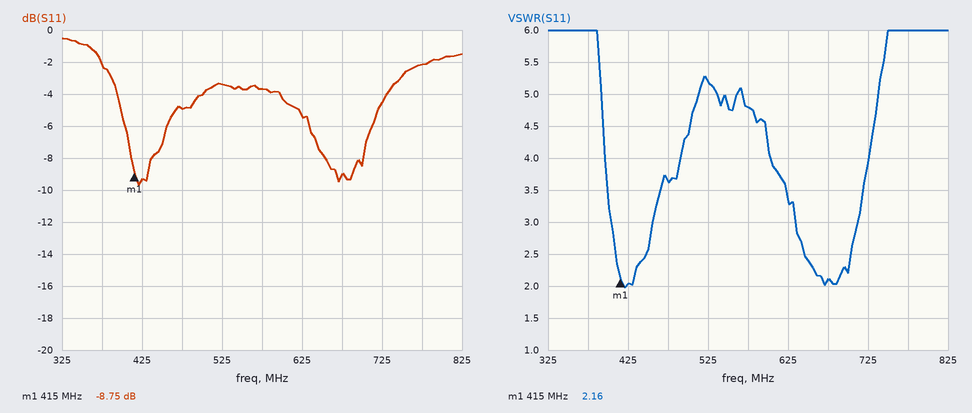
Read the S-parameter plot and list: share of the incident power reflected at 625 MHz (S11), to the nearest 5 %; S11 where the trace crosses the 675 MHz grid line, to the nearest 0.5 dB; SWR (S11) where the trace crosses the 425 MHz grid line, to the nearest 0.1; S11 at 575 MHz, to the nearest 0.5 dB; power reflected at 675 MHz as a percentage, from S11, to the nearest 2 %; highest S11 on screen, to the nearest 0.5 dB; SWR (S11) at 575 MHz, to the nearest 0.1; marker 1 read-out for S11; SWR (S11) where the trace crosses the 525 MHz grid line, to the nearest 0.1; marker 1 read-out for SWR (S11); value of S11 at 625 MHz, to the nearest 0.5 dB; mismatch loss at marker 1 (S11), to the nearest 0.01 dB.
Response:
30 %
-9.0 dB
2.0
-3.5 dB
12 %
-0.5 dB
4.8
-8.75 dB
5.2
2.16
-5.5 dB
0.62 dB
